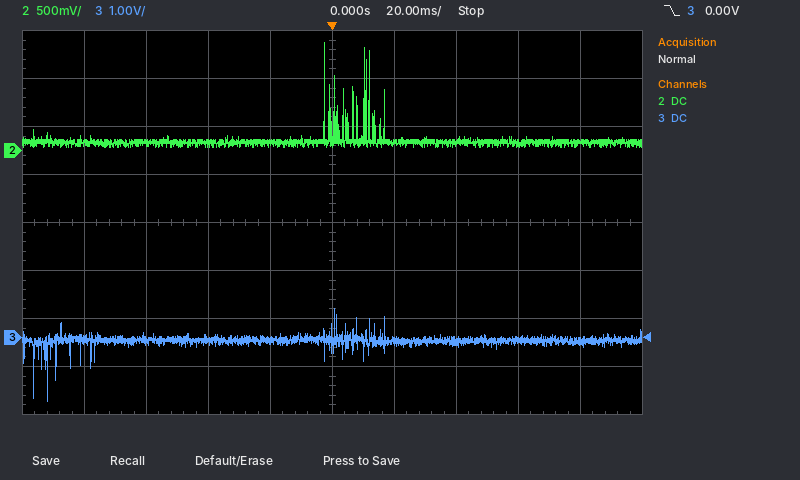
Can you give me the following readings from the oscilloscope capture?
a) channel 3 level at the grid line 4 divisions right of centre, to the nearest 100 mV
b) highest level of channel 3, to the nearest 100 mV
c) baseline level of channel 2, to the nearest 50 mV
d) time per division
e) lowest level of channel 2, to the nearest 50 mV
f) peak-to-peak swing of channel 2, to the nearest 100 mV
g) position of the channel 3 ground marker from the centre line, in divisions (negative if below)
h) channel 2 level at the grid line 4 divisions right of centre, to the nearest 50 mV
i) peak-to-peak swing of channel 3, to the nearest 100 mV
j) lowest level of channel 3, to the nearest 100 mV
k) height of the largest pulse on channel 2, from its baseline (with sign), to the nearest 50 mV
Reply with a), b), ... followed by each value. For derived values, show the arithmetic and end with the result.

a) -100 mV
b) 600 mV
c) 100 mV
d) 20 ms
e) 50 mV
f) 1.10 V
g) -2.4 div
h) 100 mV
i) 600 mV − (-1.3 V) = 1.9 V
j) -1.3 V
k) +1.05 V
